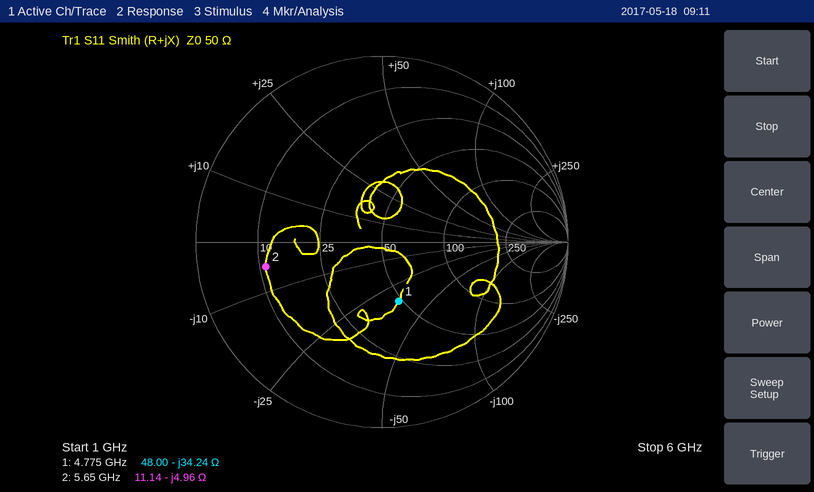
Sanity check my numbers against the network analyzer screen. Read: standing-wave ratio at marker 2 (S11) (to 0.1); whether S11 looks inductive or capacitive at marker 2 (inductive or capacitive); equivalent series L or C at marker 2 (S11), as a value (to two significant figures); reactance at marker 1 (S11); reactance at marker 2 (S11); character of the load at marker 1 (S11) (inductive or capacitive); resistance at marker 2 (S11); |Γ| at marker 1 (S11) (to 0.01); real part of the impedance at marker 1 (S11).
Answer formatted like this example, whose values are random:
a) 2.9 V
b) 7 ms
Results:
a) 4.5
b) capacitive
c) 5.7 pF
d) -34.24 Ω
e) -4.96 Ω
f) capacitive
g) 11.14 Ω
h) 0.33
i) 48.00 Ω
